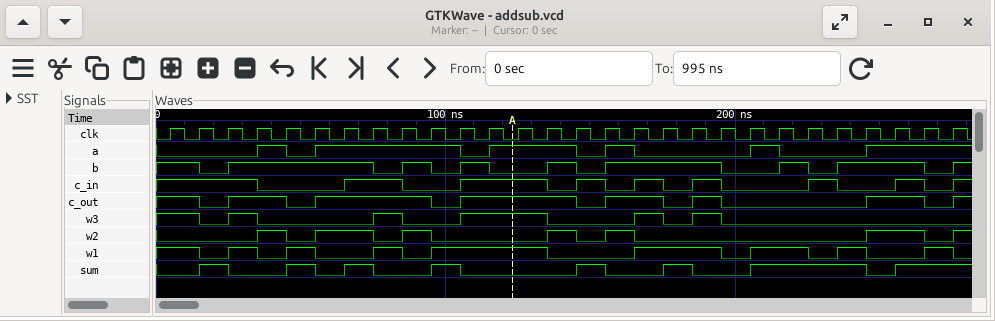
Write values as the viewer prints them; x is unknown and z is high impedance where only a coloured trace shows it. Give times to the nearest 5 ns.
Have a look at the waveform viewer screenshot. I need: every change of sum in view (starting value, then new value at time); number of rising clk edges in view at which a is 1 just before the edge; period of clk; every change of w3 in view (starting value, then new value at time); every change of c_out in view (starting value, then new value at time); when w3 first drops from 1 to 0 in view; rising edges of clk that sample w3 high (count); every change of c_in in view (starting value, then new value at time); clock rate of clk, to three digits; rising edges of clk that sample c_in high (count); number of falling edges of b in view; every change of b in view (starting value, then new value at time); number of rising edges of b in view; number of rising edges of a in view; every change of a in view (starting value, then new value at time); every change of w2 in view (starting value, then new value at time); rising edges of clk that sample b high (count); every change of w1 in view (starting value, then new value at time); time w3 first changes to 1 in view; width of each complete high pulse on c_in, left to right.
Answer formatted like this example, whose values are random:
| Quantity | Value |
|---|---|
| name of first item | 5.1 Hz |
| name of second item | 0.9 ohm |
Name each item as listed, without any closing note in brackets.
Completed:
| Quantity | Value |
|---|---|
| every change of sum in view | 0, 1 at 15 ns, 0 at 25 ns, 1 at 45 ns, 0 at 55 ns, 1 at 65 ns, 0 at 75 ns, 1 at 95 ns, 0 at 105 ns, 1 at 145 ns, 0 at 155 ns, 1 at 175 ns, 0 at 185 ns, 1 at 205 ns, 0 at 245 ns, 1 at 255 ns |
| number of rising clk edges in view at which a is 1 just before the edge | 14 |
| period of clk | 10 ns |
| every change of w3 in view | 1, 0 at 15 ns, 1 at 25 ns, 0 at 35 ns, 1 at 75 ns, 0 at 85 ns, 1 at 105 ns, 0 at 135 ns, 1 at 165 ns, 0 at 175 ns, 1 at 185 ns, 0 at 195 ns |
| every change of c_out in view | 1, 0 at 15 ns, 1 at 25 ns, 0 at 45 ns, 1 at 55 ns, 0 at 95 ns, 1 at 105 ns, 0 at 145 ns, 1 at 155 ns, 0 at 175 ns, 1 at 185 ns, 0 at 195 ns, 1 at 245 ns, 0 at 265 ns, 1 at 275 ns |
| when w3 first drops from 1 to 0 in view | 15 ns |
| rising edges of clk that sample w3 high | 9 |
| every change of c_in in view | 1, 0 at 35 ns, 1 at 65 ns, 0 at 85 ns, 1 at 105 ns, 0 at 135 ns, 1 at 145 ns, 0 at 155 ns, 1 at 165 ns, 0 at 175 ns, 1 at 185 ns, 0 at 195 ns, 1 at 225 ns, 0 at 235 ns, 1 at 255 ns, 0 at 265 ns, 1 at 275 ns |
| clock rate of clk, to three digits | 100 MHz |
| rising edges of clk that sample c_in high | 14 |
| number of falling edges of b in view | 8 |
| every change of b in view | 1, 0 at 15 ns, 1 at 25 ns, 0 at 75 ns, 1 at 85 ns, 0 at 95 ns, 1 at 105 ns, 0 at 115 ns, 1 at 135 ns, 0 at 145 ns, 1 at 155 ns, 0 at 195 ns, 1 at 215 ns, 0 at 225 ns, 1 at 235 ns, 0 at 265 ns, 1 at 275 ns |
| number of rising edges of b in view | 8 |
| number of rising edges of a in view | 6 |
| every change of a in view | 0, 1 at 35 ns, 0 at 45 ns, 1 at 55 ns, 0 at 105 ns, 1 at 115 ns, 0 at 145 ns, 1 at 155 ns, 0 at 165 ns, 1 at 205 ns, 0 at 215 ns, 1 at 245 ns |
| every change of w2 in view | 0, 1 at 35 ns, 0 at 45 ns, 1 at 55 ns, 0 at 75 ns, 1 at 85 ns, 0 at 95 ns, 1 at 135 ns, 0 at 145 ns, 1 at 155 ns, 0 at 165 ns, 1 at 245 ns, 0 at 265 ns, 1 at 275 ns |
| rising edges of clk that sample b high | 18 |
| every change of w1 in view | 1, 0 at 15 ns, 1 at 25 ns, 0 at 35 ns, 1 at 45 ns, 0 at 55 ns, 1 at 75 ns, 0 at 85 ns, 1 at 95 ns, 0 at 135 ns, 1 at 165 ns, 0 at 195 ns, 1 at 205 ns, 0 at 225 ns, 1 at 235 ns, 0 at 245 ns, 1 at 265 ns, 0 at 275 ns |
| time w3 first changes to 1 in view | 25 ns |
| width of each complete high pulse on c_in, left to right | 20 ns, 30 ns, 10 ns, 10 ns, 10 ns, 10 ns, 10 ns |
